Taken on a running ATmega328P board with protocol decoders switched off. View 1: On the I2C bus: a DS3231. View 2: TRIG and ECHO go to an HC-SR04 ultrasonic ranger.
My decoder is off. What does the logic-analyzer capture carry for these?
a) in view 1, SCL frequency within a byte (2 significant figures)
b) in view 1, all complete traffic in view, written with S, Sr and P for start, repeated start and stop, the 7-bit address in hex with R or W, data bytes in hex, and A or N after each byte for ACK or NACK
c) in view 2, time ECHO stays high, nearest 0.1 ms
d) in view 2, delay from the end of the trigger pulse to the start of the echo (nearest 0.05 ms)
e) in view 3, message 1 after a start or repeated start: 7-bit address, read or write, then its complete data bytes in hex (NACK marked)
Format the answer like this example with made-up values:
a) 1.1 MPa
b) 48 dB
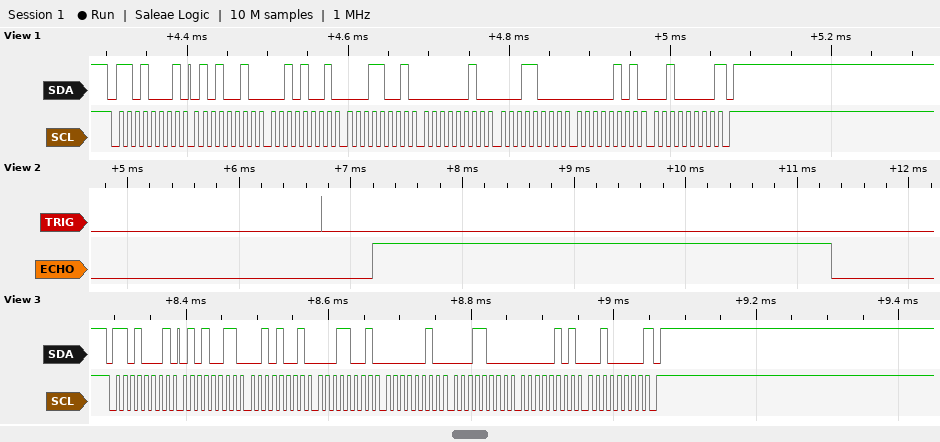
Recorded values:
a) 100 kHz
b) S 68R A 52 A 29 A 19 A 02 A 18 A 05 A 20 N P
c) 4.1 ms
d) 0.45 ms
e) 0x68 read: 53 29 19 02 18 05 20 NACK
